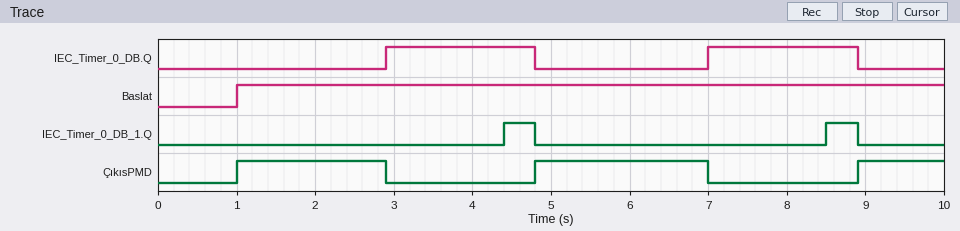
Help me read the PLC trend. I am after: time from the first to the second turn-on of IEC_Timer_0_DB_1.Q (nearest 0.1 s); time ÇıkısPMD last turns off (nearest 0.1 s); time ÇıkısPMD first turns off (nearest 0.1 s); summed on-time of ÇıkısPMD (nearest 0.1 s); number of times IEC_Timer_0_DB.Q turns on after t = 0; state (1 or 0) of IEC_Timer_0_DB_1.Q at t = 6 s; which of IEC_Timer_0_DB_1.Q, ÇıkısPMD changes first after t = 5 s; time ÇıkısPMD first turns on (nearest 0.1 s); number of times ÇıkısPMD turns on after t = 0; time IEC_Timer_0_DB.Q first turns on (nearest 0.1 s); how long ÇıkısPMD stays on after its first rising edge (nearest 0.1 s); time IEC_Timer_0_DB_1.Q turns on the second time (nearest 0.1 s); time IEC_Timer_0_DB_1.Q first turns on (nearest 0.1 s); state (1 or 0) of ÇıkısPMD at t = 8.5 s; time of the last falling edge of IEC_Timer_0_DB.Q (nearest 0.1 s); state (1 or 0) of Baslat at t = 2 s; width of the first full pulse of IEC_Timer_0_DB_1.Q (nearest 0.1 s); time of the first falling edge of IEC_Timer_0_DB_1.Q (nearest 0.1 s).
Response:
4.1 s
7.0 s
2.9 s
5.2 s
2
0
ÇıkısPMD
1.0 s
3
2.9 s
1.9 s
8.5 s
4.4 s
0
8.9 s
1
0.4 s
4.8 s
